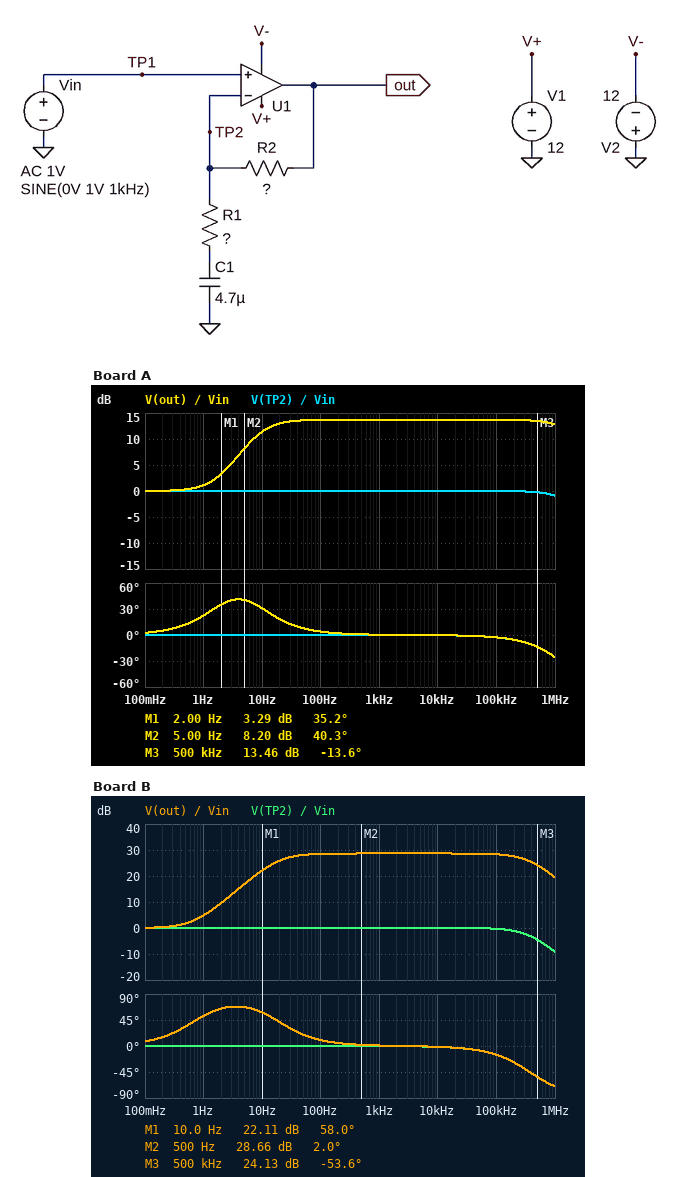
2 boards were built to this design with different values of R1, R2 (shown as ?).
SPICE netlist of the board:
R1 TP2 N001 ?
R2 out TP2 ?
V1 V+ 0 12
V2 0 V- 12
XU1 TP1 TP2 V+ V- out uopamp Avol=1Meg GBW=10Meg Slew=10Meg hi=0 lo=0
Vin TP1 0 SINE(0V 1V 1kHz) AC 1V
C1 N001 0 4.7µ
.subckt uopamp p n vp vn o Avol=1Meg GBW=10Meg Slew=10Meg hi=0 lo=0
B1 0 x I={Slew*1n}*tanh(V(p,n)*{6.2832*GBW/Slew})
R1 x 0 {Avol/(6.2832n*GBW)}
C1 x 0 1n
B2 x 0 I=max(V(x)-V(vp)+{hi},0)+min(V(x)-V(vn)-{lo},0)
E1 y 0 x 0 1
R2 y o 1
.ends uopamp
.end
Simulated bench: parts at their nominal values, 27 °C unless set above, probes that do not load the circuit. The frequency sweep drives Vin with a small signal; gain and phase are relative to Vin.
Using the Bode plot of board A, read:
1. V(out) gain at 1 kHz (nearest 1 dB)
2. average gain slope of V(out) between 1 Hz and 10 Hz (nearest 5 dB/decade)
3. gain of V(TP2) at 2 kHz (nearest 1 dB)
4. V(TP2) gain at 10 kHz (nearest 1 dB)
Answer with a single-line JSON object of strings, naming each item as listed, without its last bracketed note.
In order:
{"V(out) gain at 1 kHz": "14 dB", "average gain slope of V(out) between 1 Hz and 10 Hz": "10 dB/decade", "gain of V(TP2) at 2 kHz": "0 dB", "V(TP2) gain at 10 kHz": "0 dB"}
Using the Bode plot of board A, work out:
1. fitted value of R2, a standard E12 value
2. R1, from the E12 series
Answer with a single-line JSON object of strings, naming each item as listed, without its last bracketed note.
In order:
{"fitted value of R2, a standard E12 value": "15 kΩ", "R1, from the E12 series": "3.9 kΩ"}
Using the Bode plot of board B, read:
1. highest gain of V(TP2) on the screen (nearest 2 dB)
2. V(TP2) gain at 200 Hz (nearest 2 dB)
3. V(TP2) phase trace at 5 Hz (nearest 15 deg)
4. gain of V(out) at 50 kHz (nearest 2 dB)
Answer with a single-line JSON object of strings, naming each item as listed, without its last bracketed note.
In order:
{"highest gain of V(TP2) on the screen": "0 dB", "V(TP2) gain at 200 Hz": "0 dB", "V(TP2) phase trace at 5 Hz": "0 deg", "gain of V(out) at 50 kHz": "28 dB"}
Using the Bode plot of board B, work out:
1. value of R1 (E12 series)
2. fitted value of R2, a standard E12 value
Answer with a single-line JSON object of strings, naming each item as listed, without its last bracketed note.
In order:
{"value of R1": "1.8 kΩ", "fitted value of R2, a standard E12 value": "47 kΩ"}
